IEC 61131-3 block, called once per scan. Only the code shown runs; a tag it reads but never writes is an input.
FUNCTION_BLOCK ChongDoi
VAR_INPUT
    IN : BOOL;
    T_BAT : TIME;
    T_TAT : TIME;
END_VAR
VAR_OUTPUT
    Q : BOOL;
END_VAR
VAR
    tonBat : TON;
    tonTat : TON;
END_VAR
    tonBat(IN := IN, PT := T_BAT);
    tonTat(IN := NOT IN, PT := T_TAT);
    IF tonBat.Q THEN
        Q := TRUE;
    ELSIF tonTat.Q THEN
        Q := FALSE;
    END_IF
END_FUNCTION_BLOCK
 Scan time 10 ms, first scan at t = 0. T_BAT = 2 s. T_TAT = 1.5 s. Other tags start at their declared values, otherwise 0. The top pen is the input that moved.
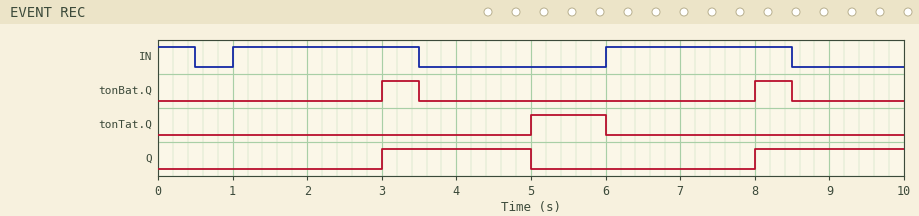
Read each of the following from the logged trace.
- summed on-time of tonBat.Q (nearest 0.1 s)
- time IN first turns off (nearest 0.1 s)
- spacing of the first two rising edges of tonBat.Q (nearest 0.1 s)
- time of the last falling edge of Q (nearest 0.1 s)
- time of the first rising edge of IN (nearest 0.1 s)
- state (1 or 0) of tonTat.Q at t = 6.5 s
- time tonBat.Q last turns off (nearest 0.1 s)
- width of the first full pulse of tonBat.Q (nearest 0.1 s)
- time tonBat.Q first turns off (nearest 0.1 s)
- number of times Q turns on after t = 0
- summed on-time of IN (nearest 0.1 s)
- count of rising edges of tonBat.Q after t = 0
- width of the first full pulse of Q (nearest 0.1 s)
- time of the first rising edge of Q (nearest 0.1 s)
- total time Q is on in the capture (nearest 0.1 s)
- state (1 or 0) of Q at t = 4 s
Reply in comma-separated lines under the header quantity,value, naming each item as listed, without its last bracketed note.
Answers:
quantity,value
summed on-time of tonBat.Q,1.0 s
time IN first turns off,0.5 s
spacing of the first two rising edges of tonBat.Q,5.0 s
time of the last falling edge of Q,5.0 s
time of the first rising edge of IN,1.0 s
state (1 or 0) of tonTat.Q at t = 6.5 s,0
time tonBat.Q last turns off,8.5 s
width of the first full pulse of tonBat.Q,0.5 s
time tonBat.Q first turns off,3.5 s
number of times Q turns on after t = 0,2
summed on-time of IN,5.5 s
count of rising edges of tonBat.Q after t = 0,2
width of the first full pulse of Q,2.0 s
time of the first rising edge of Q,3.0 s
total time Q is on in the capture,4.0 s
state (1 or 0) of Q at t = 4 s,1
